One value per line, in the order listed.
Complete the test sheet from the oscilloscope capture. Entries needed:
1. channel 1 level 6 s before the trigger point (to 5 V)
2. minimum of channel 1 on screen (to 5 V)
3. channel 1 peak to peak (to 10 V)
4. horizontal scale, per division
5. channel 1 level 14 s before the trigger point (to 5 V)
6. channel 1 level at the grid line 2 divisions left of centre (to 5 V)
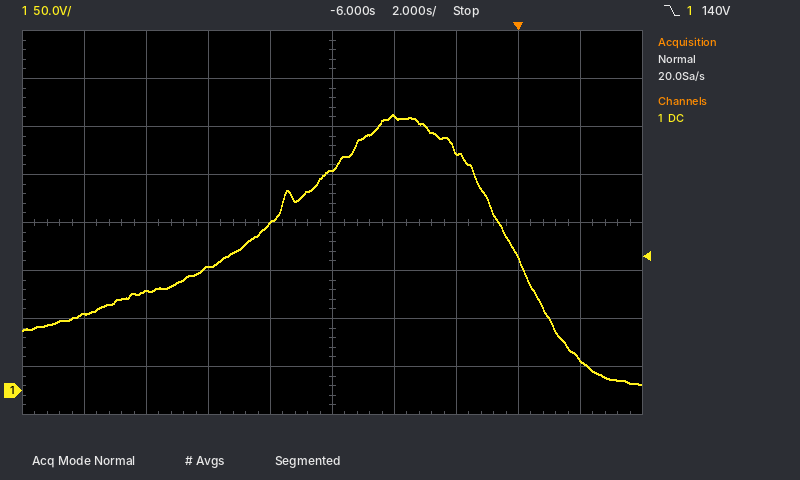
230 V
5 V
280 V
2 s
80 V
130 V
